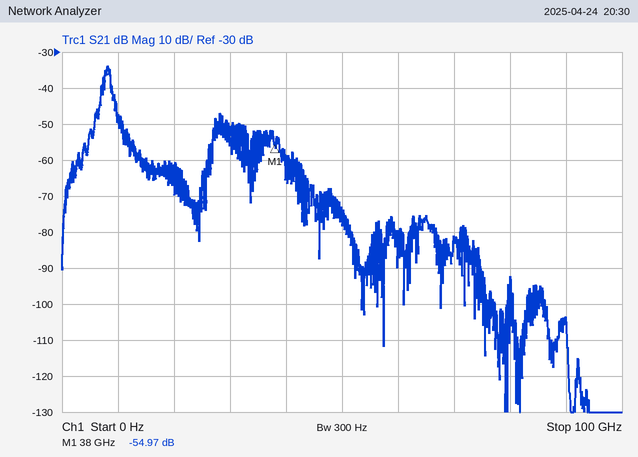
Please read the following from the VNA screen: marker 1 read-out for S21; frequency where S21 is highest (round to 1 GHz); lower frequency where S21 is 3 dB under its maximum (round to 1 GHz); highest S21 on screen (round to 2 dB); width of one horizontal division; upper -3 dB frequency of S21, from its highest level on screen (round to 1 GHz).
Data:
-54.97 dB
8 GHz
8 GHz
-34 dB
10 GHz
9 GHz
